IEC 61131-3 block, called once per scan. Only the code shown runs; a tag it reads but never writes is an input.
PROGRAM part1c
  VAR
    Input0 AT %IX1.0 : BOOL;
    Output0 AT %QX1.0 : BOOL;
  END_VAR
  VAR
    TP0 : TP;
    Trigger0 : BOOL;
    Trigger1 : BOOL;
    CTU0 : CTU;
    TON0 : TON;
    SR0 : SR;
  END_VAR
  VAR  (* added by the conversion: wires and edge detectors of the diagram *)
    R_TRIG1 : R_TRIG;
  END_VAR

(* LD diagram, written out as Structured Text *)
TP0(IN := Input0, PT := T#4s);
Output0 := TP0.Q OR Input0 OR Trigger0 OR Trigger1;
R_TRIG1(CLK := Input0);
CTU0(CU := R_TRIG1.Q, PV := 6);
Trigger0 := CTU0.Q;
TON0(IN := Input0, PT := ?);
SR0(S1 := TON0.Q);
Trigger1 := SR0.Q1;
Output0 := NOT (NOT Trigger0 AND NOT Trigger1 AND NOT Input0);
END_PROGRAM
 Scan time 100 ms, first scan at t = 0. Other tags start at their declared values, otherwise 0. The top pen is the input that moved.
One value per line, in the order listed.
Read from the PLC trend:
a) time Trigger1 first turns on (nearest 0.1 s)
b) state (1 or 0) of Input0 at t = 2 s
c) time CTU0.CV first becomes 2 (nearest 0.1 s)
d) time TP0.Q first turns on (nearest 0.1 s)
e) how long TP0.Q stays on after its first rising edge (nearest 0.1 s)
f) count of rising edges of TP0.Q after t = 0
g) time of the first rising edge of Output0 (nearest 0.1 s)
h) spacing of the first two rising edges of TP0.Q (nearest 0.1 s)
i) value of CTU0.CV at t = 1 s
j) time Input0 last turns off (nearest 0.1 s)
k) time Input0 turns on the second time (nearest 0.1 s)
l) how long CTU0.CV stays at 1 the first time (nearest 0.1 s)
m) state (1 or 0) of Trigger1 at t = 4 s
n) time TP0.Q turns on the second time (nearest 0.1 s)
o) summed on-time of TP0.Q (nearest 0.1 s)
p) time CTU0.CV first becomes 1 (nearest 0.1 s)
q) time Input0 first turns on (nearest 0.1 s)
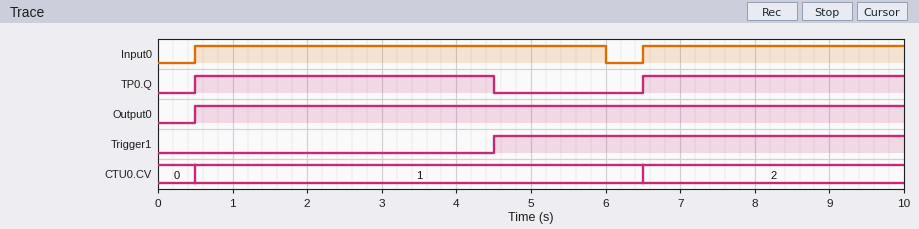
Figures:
4.5 s
1
6.5 s
0.5 s
4.0 s
2
0.5 s
6.0 s
1
6.0 s
6.5 s
6.0 s
0
6.5 s
7.5 s
0.5 s
0.5 s
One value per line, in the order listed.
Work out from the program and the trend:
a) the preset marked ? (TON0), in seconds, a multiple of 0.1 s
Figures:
4.0 s
